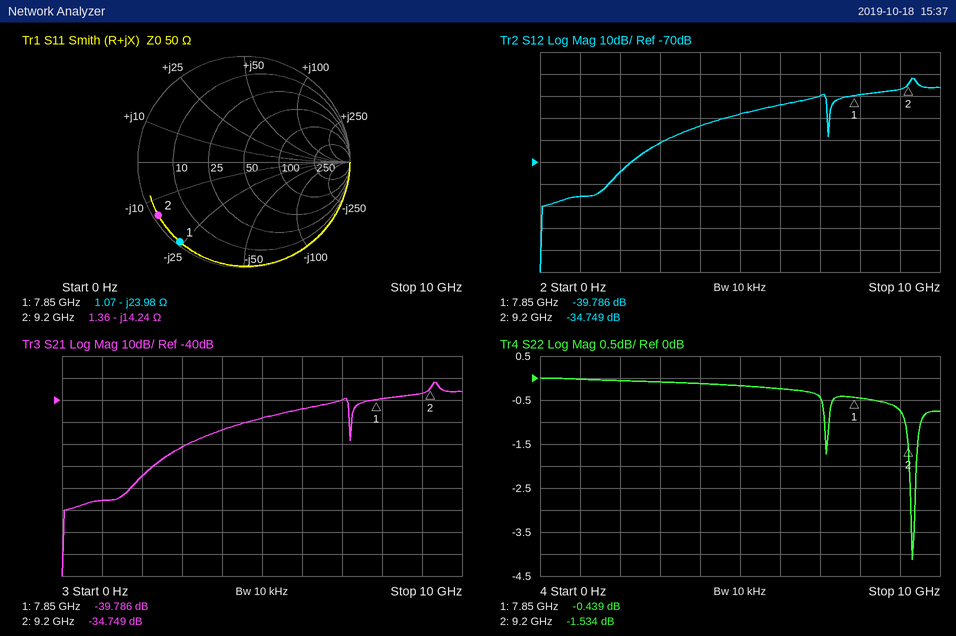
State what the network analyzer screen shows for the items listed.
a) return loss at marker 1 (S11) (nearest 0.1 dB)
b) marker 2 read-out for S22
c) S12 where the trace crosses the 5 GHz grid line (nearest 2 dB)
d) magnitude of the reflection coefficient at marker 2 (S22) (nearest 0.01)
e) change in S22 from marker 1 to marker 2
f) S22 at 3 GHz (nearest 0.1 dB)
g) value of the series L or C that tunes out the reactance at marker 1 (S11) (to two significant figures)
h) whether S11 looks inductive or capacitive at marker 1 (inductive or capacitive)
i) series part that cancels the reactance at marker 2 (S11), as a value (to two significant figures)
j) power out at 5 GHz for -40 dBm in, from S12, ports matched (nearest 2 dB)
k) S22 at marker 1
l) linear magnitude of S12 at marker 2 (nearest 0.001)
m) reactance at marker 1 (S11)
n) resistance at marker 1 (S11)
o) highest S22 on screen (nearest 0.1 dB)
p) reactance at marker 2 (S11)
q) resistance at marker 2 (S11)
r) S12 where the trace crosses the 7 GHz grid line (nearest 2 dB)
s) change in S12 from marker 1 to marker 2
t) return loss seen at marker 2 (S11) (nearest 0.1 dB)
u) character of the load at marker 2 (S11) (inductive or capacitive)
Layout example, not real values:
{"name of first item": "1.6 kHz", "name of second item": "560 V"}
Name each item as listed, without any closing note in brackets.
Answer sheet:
{"return loss at marker 1 (S11)": "0.3 dB", "marker 2 read-out for S22": "-1.534 dB", "S12 where the trace crosses the 5 GHz grid line": "-48 dB", "magnitude of the reflection coefficient at marker 2 (S22)": "0.84", "change in S22 from marker 1 to marker 2": "-1.095 dB", "S22 at 3 GHz": "-0.1 dB", "value of the series L or C that tunes out the reactance at marker 1 (S11)": "490 pH", "whether S11 looks inductive or capacitive at marker 1": "capacitive", "series part that cancels the reactance at marker 2 (S11), as a value": "250 pH", "power out at 5 GHz for -40 dBm in, from S12, ports matched": "-88 dBm", "S22 at marker 1": "-0.439 dB", "linear magnitude of S12 at marker 2": "0.018", "reactance at marker 1": "-23.98 Ω", "resistance at marker 1": "1.07 Ω", "highest S22 on screen": "0.0 dB", "reactance at marker 2": "-14.24 Ω", "resistance at marker 2": "1.36 Ω", "S12 where the trace crosses the 7 GHz grid line": "-40 dB", "change in S12 from marker 1 to marker 2": "5.037 dB", "return loss seen at marker 2 (S11)": "0.4 dB", "character of the load at marker 2 (S11)": "capacitive"}
